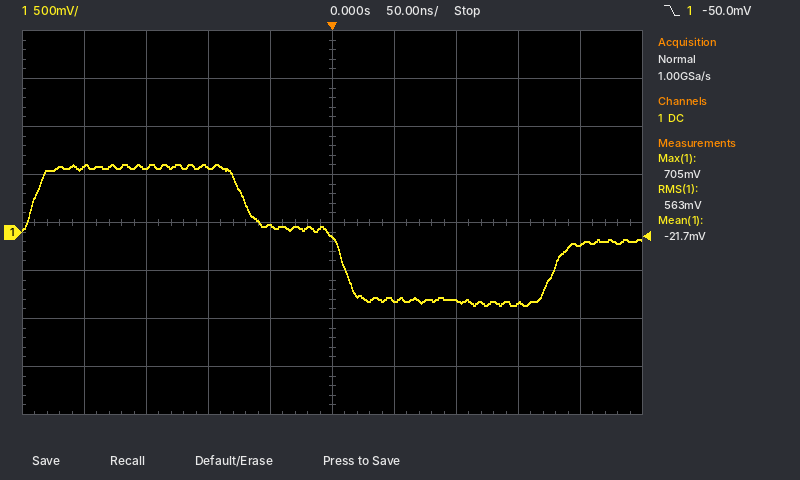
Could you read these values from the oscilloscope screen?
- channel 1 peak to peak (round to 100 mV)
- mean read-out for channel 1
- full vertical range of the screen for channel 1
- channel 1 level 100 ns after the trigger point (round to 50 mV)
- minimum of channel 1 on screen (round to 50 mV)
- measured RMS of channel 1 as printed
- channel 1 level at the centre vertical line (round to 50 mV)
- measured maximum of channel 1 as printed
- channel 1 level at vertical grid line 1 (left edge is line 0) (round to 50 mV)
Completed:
1.50 V
-21.7 mV
4 V
-700 mV
-750 mV
563 mV
-50 mV
705 mV
700 mV
